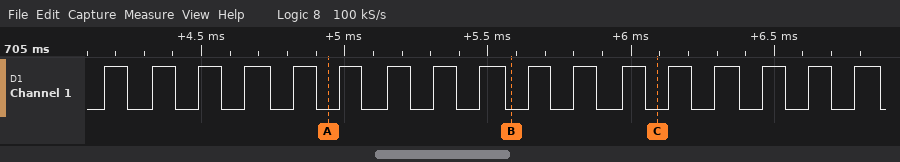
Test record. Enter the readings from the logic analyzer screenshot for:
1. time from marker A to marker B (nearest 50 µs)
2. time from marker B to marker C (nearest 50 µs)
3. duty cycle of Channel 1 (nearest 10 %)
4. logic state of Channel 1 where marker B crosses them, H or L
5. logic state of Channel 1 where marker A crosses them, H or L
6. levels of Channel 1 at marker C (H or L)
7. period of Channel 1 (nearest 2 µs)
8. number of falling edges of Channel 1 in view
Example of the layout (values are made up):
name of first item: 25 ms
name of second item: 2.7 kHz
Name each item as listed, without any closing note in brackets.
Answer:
time from marker A to marker B: 650 µs
time from marker B to marker C: 500 µs
duty cycle of Channel 1: 50 %
logic state of Channel 1 where marker B crosses them, H or L: Channel 1=L
logic state of Channel 1 where marker A crosses them, H or L: Channel 1=L
levels of Channel 1 at marker C: Channel 1=L
period of Channel 1: 164 µs
number of falling edges of Channel 1 in view: 17
